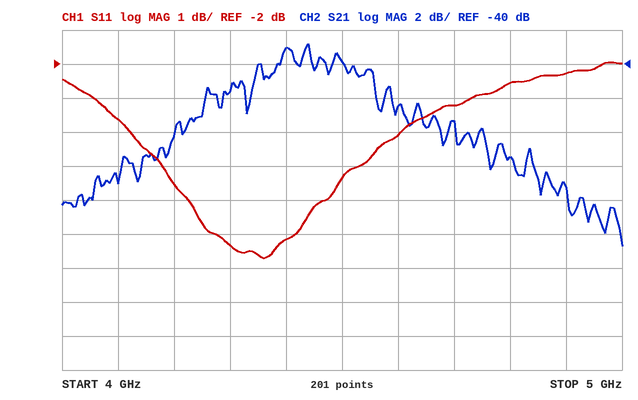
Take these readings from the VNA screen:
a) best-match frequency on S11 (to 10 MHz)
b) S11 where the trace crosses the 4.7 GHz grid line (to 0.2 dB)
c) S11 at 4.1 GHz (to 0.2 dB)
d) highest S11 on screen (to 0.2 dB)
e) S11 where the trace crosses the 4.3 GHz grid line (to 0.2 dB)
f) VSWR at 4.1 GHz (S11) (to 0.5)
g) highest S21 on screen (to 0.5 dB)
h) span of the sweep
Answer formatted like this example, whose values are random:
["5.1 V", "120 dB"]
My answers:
["4.36 GHz", "-3.2 dB", "-3.6 dB", "-2.0 dB", "-7.4 dB", "5.0", "-39.0 dB", "1 GHz"]
